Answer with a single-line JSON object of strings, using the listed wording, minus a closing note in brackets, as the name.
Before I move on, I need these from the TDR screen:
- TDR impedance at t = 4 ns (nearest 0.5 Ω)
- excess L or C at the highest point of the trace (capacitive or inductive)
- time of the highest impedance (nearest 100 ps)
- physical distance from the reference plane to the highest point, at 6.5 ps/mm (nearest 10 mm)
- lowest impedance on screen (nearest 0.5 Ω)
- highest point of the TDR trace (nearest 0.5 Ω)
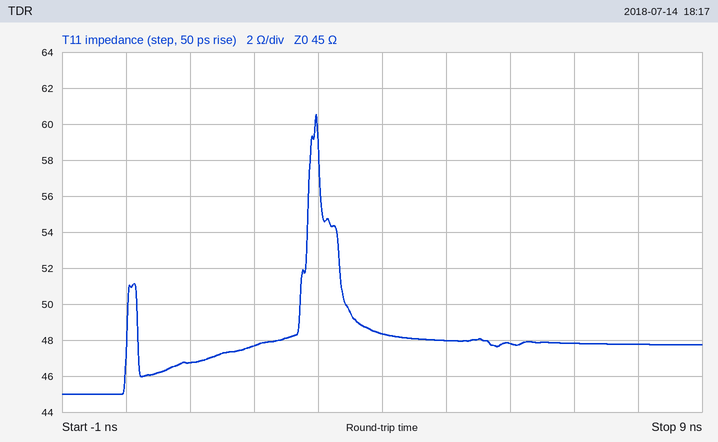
{"TDR impedance at t = 4 ns": "48.5 Ω", "excess L or C at the highest point of the trace": "inductive", "time of the highest impedance": "3.0 ns", "physical distance from the reference plane to the highest point, at 6.5 ps/mm": "230 mm", "lowest impedance on screen": "45.0 Ω", "highest point of the TDR trace": "60.5 Ω"}
